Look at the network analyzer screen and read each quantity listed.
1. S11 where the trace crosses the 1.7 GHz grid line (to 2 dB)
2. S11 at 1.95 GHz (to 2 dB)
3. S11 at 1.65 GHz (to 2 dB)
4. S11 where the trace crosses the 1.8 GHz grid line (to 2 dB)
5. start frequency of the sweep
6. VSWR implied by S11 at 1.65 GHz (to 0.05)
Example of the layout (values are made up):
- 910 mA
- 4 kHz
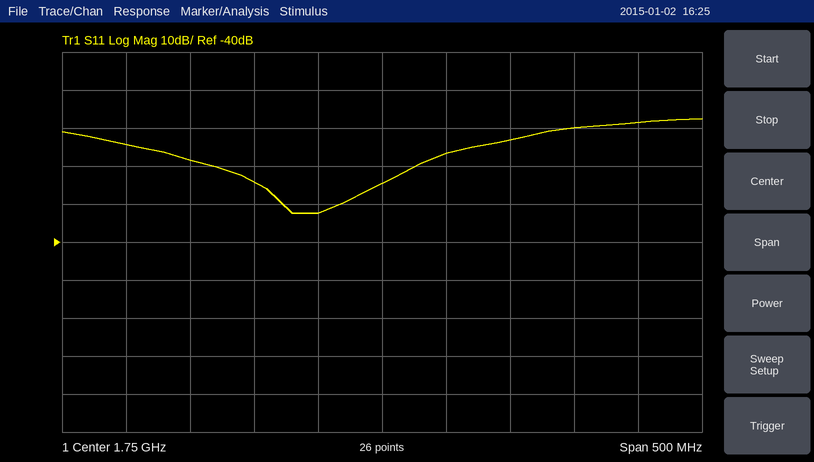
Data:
- -32 dB
- -8 dB
- -24 dB
- -16 dB
- 1.5 GHz
- 1.15
